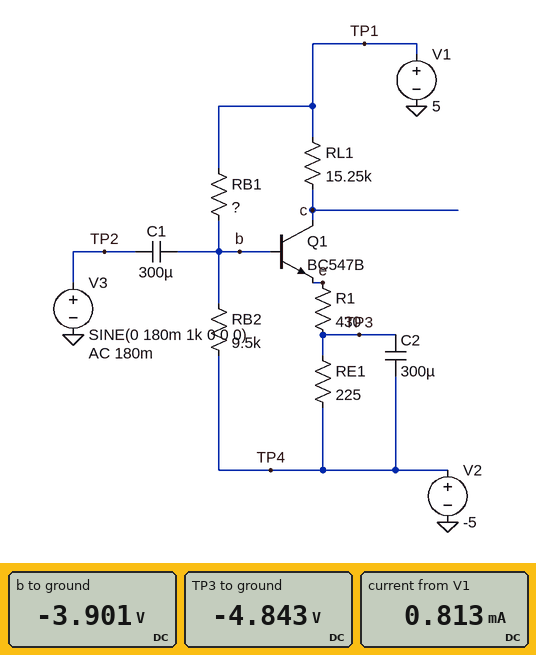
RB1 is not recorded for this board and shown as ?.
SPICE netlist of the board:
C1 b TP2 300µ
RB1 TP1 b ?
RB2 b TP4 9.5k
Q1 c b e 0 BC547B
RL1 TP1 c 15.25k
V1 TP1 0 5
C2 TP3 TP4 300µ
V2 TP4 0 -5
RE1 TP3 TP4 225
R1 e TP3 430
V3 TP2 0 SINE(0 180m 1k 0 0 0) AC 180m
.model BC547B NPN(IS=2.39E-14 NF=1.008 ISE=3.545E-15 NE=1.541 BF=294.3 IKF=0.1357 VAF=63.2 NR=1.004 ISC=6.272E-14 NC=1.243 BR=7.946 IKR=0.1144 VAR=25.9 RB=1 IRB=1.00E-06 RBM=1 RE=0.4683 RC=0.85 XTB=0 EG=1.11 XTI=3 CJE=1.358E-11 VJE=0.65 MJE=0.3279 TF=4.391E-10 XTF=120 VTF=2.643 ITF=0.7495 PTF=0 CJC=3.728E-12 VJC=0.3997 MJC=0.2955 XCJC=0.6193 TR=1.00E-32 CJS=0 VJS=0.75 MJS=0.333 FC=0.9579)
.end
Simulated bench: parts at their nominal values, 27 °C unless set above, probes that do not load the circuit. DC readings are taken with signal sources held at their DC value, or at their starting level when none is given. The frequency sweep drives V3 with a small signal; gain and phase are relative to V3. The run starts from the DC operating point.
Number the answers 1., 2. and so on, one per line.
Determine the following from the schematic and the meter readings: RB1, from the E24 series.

1. 47 kΩ
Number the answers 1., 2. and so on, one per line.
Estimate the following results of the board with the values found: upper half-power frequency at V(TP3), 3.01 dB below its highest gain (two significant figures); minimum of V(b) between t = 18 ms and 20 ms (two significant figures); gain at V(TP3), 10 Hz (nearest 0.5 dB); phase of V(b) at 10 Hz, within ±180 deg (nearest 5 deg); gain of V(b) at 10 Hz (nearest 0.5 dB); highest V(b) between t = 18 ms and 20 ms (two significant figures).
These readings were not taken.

1. 4.7 Hz
2. -4.1 V
3. -21.5 dB
4. 5 deg
5. 0 dB
6. -3.7 V
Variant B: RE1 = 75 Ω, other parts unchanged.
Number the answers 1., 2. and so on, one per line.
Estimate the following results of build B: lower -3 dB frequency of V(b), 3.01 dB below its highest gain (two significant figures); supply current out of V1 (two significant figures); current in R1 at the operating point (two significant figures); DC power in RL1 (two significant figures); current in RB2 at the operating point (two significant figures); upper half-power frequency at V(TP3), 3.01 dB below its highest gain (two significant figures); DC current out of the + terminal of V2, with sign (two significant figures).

1. 890 mHz
2. 820 µA
3. 720 µA
4. 6.1 mW
5. 110 µA
6. 9.7 Hz
7. -820 µA
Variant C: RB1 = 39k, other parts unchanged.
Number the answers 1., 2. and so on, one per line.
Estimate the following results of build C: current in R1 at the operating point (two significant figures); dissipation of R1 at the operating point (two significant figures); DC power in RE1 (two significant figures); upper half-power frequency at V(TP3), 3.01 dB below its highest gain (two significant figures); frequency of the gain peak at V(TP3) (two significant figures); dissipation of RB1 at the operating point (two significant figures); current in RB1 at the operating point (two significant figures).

1. 730 µA
2. 230 µW
3. 120 µW
4. 4.8 Hz
5. 1.6 Hz
6. 2.0 mW
7. 230 µA
